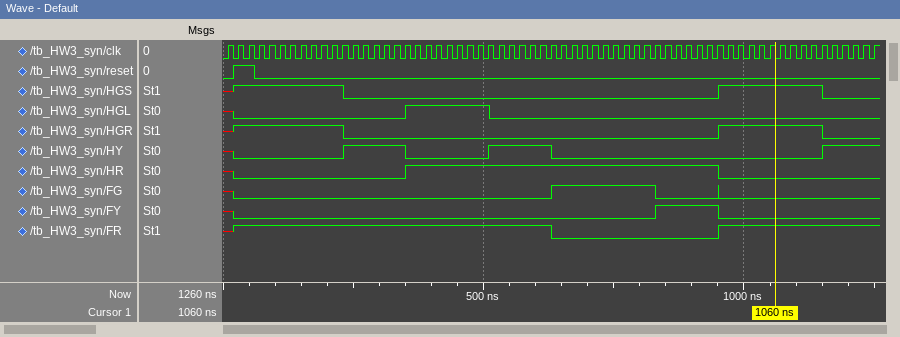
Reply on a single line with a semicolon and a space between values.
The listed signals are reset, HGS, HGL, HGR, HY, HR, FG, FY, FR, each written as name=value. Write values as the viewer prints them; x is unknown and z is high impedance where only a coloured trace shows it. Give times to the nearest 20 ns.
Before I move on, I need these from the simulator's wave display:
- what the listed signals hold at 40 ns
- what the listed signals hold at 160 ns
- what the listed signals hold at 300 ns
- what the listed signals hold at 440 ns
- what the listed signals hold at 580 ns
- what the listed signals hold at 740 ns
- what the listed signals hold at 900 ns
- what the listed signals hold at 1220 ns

reset=1, HGS=1, HGL=0, HGR=1, HY=0, HR=0, FG=0, FY=0, FR=1; reset=0, HGS=1, HGL=0, HGR=1, HY=0, HR=0, FG=0, FY=0, FR=1; reset=0, HGS=0, HGL=0, HGR=0, HY=1, HR=0, FG=0, FY=0, FR=1; reset=0, HGS=0, HGL=1, HGR=0, HY=0, HR=1, FG=0, FY=0, FR=1; reset=0, HGS=0, HGL=0, HGR=0, HY=1, HR=1, FG=0, FY=0, FR=1; reset=0, HGS=0, HGL=0, HGR=0, HY=0, HR=1, FG=1, FY=0, FR=0; reset=0, HGS=0, HGL=0, HGR=0, HY=0, HR=1, FG=0, FY=1, FR=0; reset=0, HGS=0, HGL=0, HGR=0, HY=1, HR=0, FG=0, FY=0, FR=1
